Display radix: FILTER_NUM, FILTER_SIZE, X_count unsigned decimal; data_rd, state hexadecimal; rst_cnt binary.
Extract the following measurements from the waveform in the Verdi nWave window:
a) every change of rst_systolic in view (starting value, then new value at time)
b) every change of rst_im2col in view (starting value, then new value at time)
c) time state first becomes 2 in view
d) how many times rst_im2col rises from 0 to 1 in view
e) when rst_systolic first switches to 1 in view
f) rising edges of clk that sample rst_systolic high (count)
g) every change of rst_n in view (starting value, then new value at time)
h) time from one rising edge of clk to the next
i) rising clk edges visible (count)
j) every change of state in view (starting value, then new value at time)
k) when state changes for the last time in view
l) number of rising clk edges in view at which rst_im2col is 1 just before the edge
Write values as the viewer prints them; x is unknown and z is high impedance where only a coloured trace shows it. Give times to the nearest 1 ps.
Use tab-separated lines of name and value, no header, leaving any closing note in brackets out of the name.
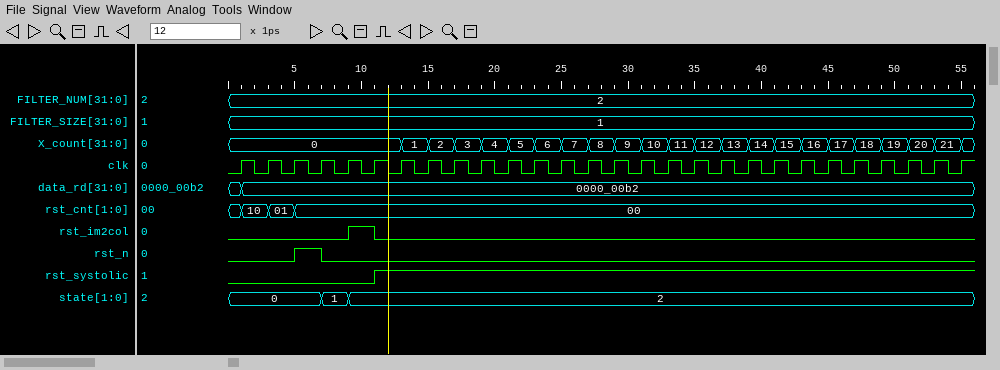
every change of rst_systolic in view	0, 1 at 11 ps
every change of rst_im2col in view	0, 1 at 9 ps, 0 at 11 ps
time state first becomes 2 in view	9 ps
how many times rst_im2col rises from 0 to 1 in view	1
when rst_systolic first switches to 1 in view	11 ps
rising edges of clk that sample rst_systolic high	22
every change of rst_n in view	0, 1 at 5 ps, 0 at 7 ps
time from one rising edge of clk to the next	2 ps
rising clk edges visible	28
every change of state in view	0, 1 at 7 ps, 2 at 9 ps
when state changes for the last time in view	9 ps
number of rising clk edges in view at which rst_im2col is 1 just before the edge	1
